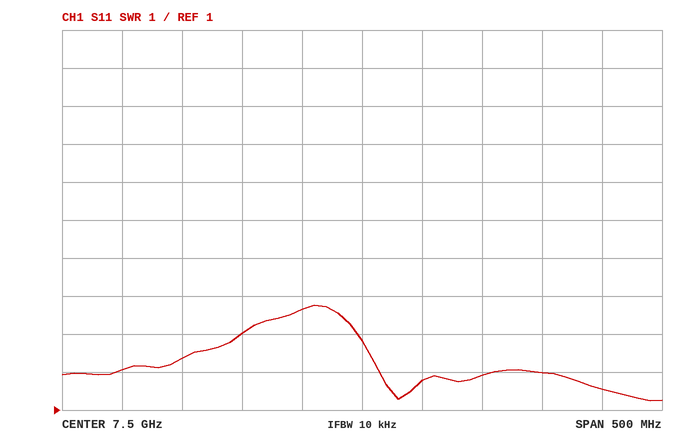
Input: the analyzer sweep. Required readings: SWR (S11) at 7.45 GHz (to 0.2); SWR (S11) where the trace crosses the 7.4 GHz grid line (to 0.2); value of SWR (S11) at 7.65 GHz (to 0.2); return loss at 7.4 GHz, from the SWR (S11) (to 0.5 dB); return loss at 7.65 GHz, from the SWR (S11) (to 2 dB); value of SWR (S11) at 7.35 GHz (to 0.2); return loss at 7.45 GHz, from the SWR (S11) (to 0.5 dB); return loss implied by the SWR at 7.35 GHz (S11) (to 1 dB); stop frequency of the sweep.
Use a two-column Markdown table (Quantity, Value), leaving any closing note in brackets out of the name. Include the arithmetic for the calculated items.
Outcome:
| Quantity | Value |
|---|---|
| SWR (S11) at 7.45 GHz | 3.6 |
| SWR (S11) where the trace crosses the 7.4 GHz grid line | 3.0 |
| value of SWR (S11) at 7.65 GHz | 2.0 |
| return loss at 7.4 GHz, from the SWR (S11) | −20 log10((3 − 1)/(3 + 1)) ≈ 6.0 dB |
| return loss at 7.65 GHz, from the SWR (S11) | −20 log10((2 − 1)/(2 + 1)) ≈ 10 dB |
| value of SWR (S11) at 7.35 GHz | 2.4 |
| return loss at 7.45 GHz, from the SWR (S11) | −20 log10((3.6 − 1)/(3.6 + 1)) ≈ 5.0 dB |
| return loss implied by the SWR at 7.35 GHz (S11) | −20 log10((2.4 − 1)/(2.4 + 1)) ≈ 8 dB |
| stop frequency of the sweep | 7.75 GHz |
